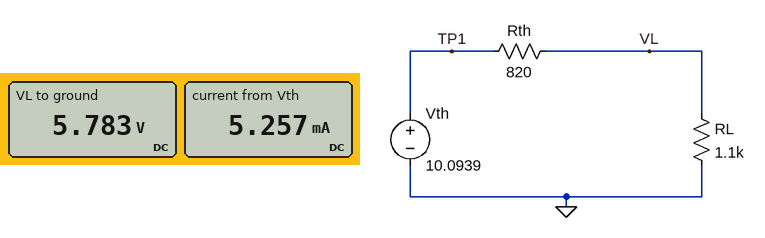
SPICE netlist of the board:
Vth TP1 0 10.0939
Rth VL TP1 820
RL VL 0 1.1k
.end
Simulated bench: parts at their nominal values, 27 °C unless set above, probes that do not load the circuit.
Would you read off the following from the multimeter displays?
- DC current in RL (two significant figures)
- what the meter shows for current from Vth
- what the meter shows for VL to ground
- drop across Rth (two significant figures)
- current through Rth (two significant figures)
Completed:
5.3 mA
5.257 mA
5.783 V
4.3 V
5.3 mA
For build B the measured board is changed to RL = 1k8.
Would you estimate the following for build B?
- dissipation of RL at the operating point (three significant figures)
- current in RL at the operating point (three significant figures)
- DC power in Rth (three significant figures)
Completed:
26.7 mW
3.85 mA
12.2 mW
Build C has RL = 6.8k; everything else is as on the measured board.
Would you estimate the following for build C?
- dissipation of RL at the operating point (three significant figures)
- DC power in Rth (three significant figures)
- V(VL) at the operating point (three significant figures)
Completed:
11.9 mW
1.44 mW
9.01 V
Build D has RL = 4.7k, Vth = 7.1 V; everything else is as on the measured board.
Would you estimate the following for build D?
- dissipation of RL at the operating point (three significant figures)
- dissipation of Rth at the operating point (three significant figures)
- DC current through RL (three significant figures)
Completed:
7.78 mW
1.36 mW
1.29 mA
